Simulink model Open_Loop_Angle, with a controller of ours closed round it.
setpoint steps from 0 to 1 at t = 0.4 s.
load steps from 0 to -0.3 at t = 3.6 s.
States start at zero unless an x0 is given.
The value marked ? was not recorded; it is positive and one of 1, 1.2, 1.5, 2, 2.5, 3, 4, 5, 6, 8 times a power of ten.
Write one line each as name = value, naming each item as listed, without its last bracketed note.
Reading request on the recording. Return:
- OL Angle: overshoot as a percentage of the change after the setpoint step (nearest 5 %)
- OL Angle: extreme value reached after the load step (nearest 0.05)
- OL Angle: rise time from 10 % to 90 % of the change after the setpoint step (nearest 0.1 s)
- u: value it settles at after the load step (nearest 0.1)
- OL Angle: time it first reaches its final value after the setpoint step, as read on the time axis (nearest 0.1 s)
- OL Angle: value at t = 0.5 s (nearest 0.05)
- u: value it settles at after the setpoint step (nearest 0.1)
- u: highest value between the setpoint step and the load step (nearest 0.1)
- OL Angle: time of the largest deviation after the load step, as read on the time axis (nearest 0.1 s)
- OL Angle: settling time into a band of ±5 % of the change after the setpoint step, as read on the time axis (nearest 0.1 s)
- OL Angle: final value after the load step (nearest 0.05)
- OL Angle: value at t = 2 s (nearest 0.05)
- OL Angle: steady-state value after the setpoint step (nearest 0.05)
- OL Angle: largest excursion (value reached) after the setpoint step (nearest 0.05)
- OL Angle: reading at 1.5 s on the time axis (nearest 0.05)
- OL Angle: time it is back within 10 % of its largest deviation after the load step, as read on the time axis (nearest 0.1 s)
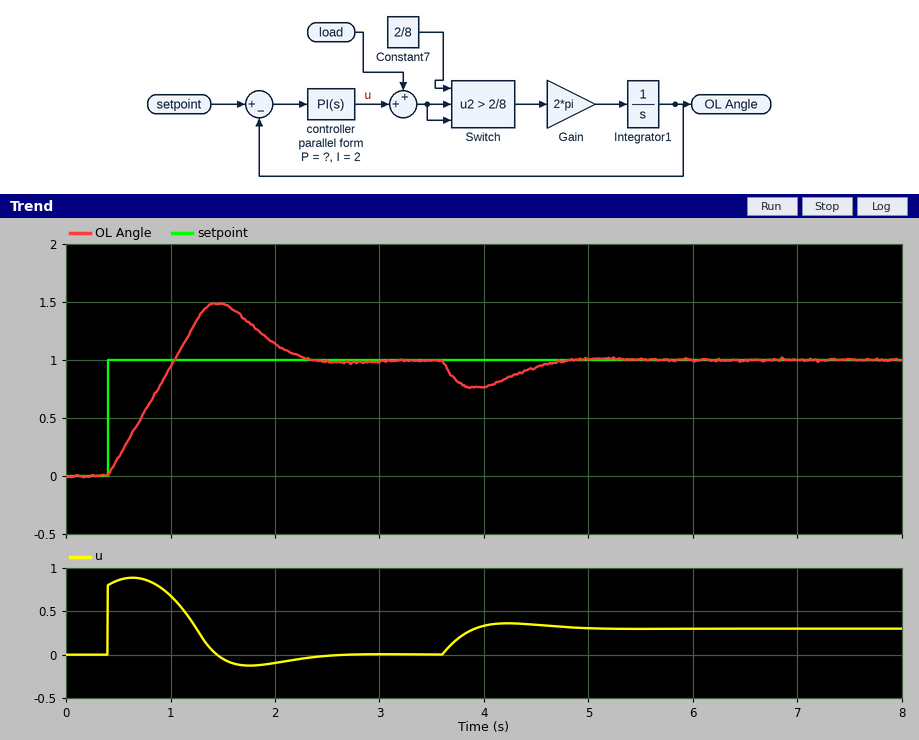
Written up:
OL Angle: overshoot as a percentage of the change after the setpoint step = 50 %
OL Angle: extreme value reached after the load step = 0.75
OL Angle: rise time from 10 % to 90 % of the change after the setpoint step = 0.5 s
u: value it settles at after the load step = 0.3
OL Angle: time it first reaches its final value after the setpoint step, as read on the time axis = 1.0 s
OL Angle: value at t = 0.5 s = 0.15
u: value it settles at after the setpoint step = 0.0
u: highest value between the setpoint step and the load step = 0.9
OL Angle: time of the largest deviation after the load step, as read on the time axis = 3.9 s
OL Angle: settling time into a band of ±5 % of the change after the setpoint step, as read on the time axis = 2.2 s
OL Angle: final value after the load step = 1.00
OL Angle: value at t = 2 s = 1.15
OL Angle: steady-state value after the setpoint step = 1.00
OL Angle: largest excursion (value reached) after the setpoint step = 1.50
OL Angle: reading at 1.5 s on the time axis = 1.50
OL Angle: time it is back within 10 % of its largest deviation after the load step, as read on the time axis = 4.7 s
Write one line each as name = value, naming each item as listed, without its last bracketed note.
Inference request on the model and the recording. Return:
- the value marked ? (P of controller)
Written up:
the value marked ? = 0.8
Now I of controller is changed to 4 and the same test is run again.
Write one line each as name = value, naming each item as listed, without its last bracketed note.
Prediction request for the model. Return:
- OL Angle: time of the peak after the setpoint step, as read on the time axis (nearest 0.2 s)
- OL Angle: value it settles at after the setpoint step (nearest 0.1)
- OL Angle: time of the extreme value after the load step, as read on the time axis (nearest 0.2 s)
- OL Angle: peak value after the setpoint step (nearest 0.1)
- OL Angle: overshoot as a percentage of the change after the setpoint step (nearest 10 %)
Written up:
OL Angle: time of the peak after the setpoint step, as read on the time axis = 1.6 s
OL Angle: value it settles at after the setpoint step = 1.0
OL Angle: time of the extreme value after the load step, as read on the time axis = 3.8 s
OL Angle: peak value after the setpoint step = 1.7
OL Angle: overshoot as a percentage of the change after the setpoint step = 70 %
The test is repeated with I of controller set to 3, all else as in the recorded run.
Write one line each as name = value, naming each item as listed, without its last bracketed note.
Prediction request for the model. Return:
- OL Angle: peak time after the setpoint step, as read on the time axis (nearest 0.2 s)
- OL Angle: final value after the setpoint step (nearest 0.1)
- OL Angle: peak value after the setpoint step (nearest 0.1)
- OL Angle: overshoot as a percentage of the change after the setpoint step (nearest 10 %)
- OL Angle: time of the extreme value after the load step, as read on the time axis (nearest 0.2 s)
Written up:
OL Angle: peak time after the setpoint step, as read on the time axis = 1.4 s
OL Angle: final value after the setpoint step = 1.0
OL Angle: peak value after the setpoint step = 1.6
OL Angle: overshoot as a percentage of the change after the setpoint step = 60 %
OL Angle: time of the extreme value after the load step, as read on the time axis = 3.8 s
